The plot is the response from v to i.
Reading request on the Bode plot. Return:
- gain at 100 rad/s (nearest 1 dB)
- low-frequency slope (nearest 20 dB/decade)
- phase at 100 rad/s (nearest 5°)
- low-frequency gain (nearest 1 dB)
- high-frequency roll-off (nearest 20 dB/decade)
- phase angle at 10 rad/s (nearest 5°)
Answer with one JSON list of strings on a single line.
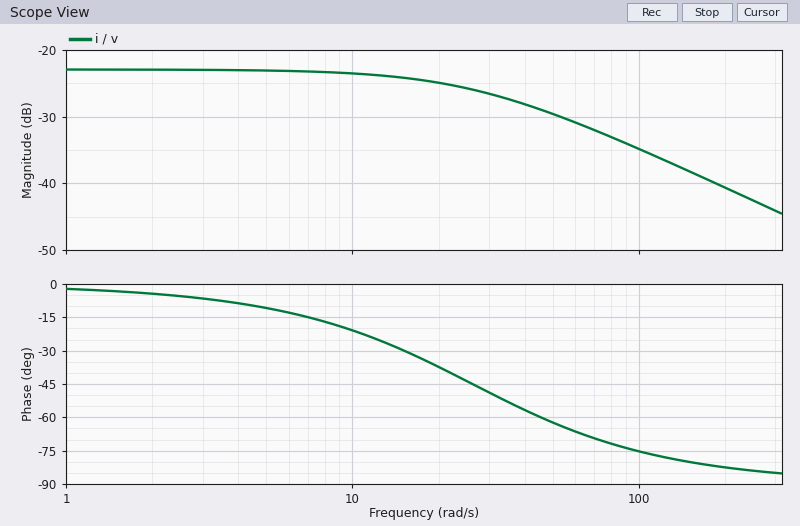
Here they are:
["-35 dB", "0 dB/decade", "-75°", "-23 dB", "-20 dB/decade", "-20°"]
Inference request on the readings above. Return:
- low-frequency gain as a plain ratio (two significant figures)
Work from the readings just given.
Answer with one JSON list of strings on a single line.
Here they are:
["0.071"]
